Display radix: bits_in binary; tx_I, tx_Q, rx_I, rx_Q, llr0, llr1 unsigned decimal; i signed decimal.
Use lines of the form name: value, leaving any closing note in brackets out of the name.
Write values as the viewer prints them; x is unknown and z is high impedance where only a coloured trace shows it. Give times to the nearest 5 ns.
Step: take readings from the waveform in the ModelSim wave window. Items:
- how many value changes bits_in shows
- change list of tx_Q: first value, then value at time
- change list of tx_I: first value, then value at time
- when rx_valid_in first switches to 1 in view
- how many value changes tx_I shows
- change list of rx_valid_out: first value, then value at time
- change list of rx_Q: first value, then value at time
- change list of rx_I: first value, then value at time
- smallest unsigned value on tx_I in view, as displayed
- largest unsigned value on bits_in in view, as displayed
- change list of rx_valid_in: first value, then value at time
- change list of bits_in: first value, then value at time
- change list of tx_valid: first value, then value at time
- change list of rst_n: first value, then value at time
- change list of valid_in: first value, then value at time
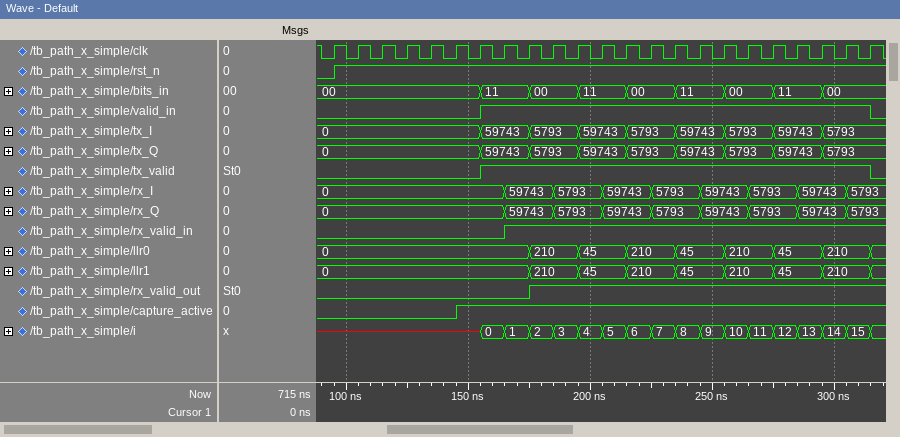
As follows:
how many value changes bits_in shows: 8
change list of tx_Q: first value, then value at time: 0, 59743 at 155 ns, 5793 at 175 ns, 59743 at 195 ns, 5793 at 215 ns, 59743 at 235 ns, 5793 at 255 ns, 59743 at 275 ns, 5793 at 295 ns
change list of tx_I: first value, then value at time: 0, 59743 at 155 ns, 5793 at 175 ns, 59743 at 195 ns, 5793 at 215 ns, 59743 at 235 ns, 5793 at 255 ns, 59743 at 275 ns, 5793 at 295 ns
when rx_valid_in first switches to 1 in view: 165 ns
how many value changes tx_I shows: 8
change list of rx_valid_out: first value, then value at time: 0, 1 at 175 ns
change list of rx_Q: first value, then value at time: 0, 59743 at 165 ns, 5793 at 185 ns, 59743 at 205 ns, 5793 at 225 ns, 59743 at 245 ns, 5793 at 265 ns, 59743 at 285 ns, 5793 at 305 ns
change list of rx_I: first value, then value at time: 0, 59743 at 165 ns, 5793 at 185 ns, 59743 at 205 ns, 5793 at 225 ns, 59743 at 245 ns, 5793 at 265 ns, 59743 at 285 ns, 5793 at 305 ns
smallest unsigned value on tx_I in view, as displayed: 0
largest unsigned value on bits_in in view, as displayed: 11
change list of rx_valid_in: first value, then value at time: 0, 1 at 165 ns
change list of bits_in: first value, then value at time: 00, 11 at 155 ns, 00 at 175 ns, 11 at 195 ns, 00 at 215 ns, 11 at 235 ns, 00 at 255 ns, 11 at 275 ns, 00 at 295 ns
change list of tx_valid: first value, then value at time: 0, 1 at 155 ns, 0 at 315 ns
change list of rst_n: first value, then value at time: 0, 1 at 95 ns
change list of valid_in: first value, then value at time: 0, 1 at 155 ns, 0 at 315 ns
